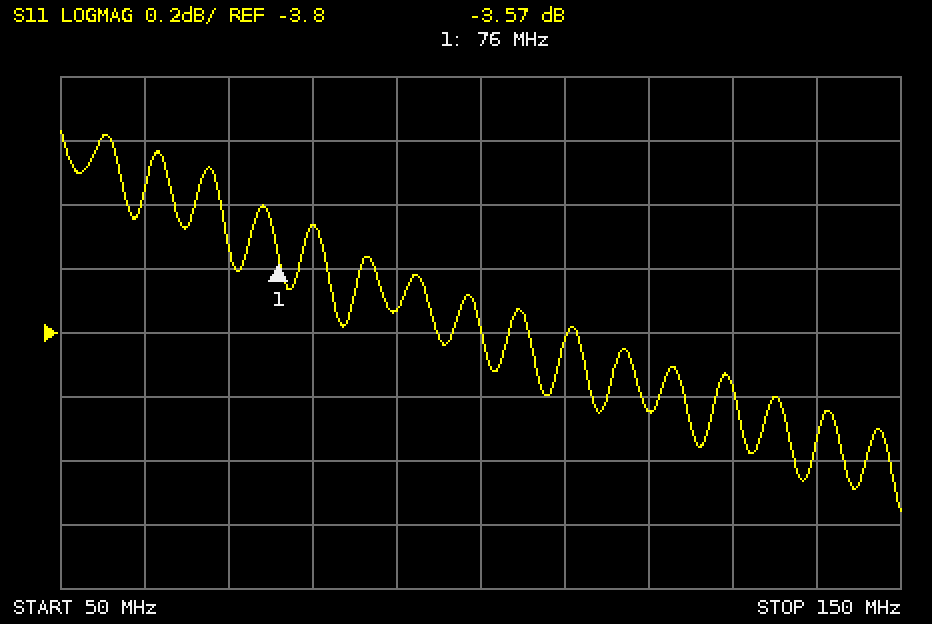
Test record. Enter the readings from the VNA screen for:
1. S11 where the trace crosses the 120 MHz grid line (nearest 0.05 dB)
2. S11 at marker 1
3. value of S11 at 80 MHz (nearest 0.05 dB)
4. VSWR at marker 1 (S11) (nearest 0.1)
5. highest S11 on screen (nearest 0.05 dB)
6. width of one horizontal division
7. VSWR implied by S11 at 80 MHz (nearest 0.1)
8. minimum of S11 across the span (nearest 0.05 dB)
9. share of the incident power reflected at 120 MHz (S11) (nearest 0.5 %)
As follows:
-4.05 dB
-3.57 dB
-3.45 dB
4.9
-3.15 dB
10 MHz
5.1
-4.35 dB
39.5 %
